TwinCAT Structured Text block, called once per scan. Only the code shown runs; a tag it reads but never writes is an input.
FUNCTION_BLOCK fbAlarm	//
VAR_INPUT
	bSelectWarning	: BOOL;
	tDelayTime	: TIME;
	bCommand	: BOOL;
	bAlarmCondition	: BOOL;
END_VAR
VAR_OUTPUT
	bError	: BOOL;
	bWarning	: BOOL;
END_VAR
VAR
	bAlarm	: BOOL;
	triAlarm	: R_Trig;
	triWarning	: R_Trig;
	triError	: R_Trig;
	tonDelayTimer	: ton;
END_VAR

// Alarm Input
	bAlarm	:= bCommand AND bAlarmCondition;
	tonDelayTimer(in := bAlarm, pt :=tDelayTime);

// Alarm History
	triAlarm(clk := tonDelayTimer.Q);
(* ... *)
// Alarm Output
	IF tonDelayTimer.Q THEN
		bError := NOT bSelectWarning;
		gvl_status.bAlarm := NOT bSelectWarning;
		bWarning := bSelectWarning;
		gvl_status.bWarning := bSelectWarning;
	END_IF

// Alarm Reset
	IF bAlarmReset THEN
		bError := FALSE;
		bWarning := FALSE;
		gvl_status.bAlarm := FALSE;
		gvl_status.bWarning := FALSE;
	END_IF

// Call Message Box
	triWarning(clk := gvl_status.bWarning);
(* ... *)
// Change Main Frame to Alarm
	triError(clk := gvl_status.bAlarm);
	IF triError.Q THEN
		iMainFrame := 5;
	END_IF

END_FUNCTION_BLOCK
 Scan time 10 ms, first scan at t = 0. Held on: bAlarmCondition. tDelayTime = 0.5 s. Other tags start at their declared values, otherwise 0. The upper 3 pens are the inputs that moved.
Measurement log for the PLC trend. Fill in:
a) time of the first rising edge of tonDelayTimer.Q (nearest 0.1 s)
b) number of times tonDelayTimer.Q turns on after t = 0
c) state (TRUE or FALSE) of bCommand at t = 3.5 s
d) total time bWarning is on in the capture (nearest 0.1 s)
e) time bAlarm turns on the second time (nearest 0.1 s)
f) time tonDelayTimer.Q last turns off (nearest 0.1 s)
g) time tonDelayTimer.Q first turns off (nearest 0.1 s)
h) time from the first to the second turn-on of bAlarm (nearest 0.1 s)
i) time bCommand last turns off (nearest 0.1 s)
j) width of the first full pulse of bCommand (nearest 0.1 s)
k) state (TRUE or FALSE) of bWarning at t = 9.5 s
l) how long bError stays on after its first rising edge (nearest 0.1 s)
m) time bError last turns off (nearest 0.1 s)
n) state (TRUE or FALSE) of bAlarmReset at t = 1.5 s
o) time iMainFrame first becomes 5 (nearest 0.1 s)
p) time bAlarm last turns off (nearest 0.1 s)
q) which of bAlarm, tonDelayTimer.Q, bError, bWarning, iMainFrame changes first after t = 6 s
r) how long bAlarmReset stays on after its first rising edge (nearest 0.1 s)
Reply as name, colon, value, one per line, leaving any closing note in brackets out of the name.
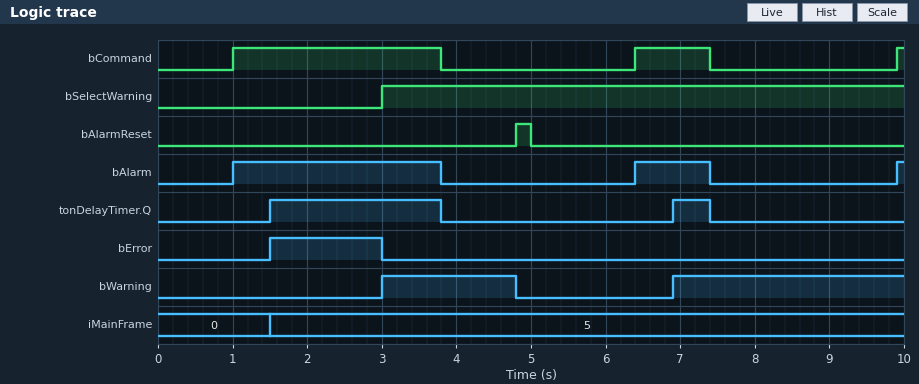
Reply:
time of the first rising edge of tonDelayTimer.Q: 1.5 s
number of times tonDelayTimer.Q turns on after t = 0: 2
state (TRUE or FALSE) of bCommand at t = 3.5 s: TRUE
total time bWarning is on in the capture: 4.9 s
time bAlarm turns on the second time: 6.4 s
time tonDelayTimer.Q last turns off: 7.4 s
time tonDelayTimer.Q first turns off: 3.8 s
time from the first to the second turn-on of bAlarm: 5.4 s
time bCommand last turns off: 7.4 s
width of the first full pulse of bCommand: 2.8 s
state (TRUE or FALSE) of bWarning at t = 9.5 s: TRUE
how long bError stays on after its first rising edge: 1.5 s
time bError last turns off: 3.0 s
state (TRUE or FALSE) of bAlarmReset at t = 1.5 s: FALSE
time iMainFrame first becomes 5: 1.5 s
time bAlarm last turns off: 7.4 s
which of bAlarm, tonDelayTimer.Q, bError, bWarning, iMainFrame changes first after t = 6 s: bAlarm
how long bAlarmReset stays on after its first rising edge: 0.2 s
